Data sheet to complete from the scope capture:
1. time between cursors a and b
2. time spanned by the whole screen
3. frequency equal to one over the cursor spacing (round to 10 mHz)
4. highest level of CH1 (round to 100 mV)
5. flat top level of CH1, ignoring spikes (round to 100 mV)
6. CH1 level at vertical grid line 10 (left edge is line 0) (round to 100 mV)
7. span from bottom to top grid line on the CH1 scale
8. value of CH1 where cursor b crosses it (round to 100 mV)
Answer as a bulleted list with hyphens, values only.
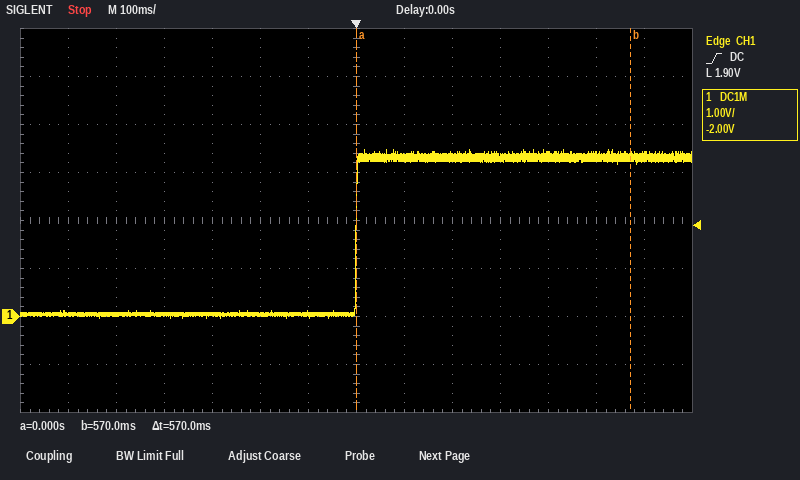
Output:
- 570 ms
- 1.4 s
- 1.75 Hz
- 3.5 V
- 3.3 V
- 3.3 V
- 8 V
- 3.3 V
